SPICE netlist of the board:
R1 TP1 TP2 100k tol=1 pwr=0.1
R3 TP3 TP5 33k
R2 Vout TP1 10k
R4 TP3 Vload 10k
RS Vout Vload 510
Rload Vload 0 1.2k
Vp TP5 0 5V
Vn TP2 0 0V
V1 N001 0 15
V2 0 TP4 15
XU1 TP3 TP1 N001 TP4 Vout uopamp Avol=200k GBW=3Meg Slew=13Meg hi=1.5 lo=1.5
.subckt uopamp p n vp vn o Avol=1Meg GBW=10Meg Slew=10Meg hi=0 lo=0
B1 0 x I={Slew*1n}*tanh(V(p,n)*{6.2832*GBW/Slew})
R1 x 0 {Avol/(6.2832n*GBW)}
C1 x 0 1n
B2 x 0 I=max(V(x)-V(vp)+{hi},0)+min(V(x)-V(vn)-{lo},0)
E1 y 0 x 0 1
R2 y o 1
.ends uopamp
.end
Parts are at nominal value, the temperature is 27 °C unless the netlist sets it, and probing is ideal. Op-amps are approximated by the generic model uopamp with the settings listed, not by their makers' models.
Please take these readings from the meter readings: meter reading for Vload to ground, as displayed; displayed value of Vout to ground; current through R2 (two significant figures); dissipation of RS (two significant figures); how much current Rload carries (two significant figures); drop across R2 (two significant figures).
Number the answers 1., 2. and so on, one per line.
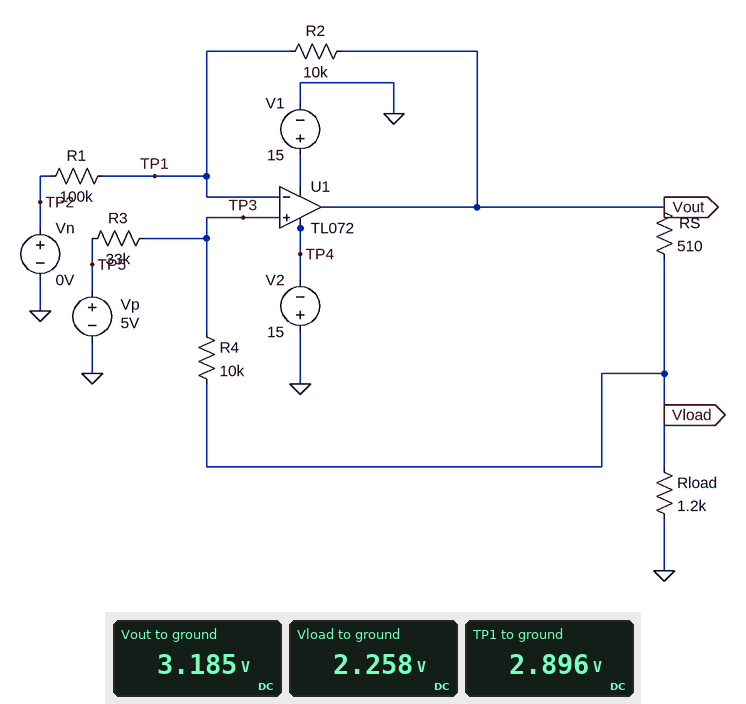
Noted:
1. 2.258 V
2. 3.185 V
3. 29 µA
4. 1.7 mW
5. 1.9 mA
6. 290 mV
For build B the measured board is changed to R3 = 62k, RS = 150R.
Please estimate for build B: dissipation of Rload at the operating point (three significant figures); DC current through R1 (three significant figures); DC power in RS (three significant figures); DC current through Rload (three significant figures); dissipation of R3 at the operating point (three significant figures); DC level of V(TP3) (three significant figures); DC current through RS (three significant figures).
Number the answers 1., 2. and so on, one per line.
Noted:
1. 15.4 mW
2. 44.0 µA
3. 1.92 mW
4. 3.59 mA
5. 5.78 µW
6. 4.40 V
7. 3.58 mA
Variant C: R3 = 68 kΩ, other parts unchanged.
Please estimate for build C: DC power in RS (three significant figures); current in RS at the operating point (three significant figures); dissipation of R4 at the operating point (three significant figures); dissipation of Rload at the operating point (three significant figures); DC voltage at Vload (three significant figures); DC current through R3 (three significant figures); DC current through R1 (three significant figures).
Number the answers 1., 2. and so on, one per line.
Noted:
1. 806 µW
2. 1.26 mA
3. 19.4 µW
4. 2.03 mW
5. 1.56 V
6. 44.1 µA
7. 20.0 µA
